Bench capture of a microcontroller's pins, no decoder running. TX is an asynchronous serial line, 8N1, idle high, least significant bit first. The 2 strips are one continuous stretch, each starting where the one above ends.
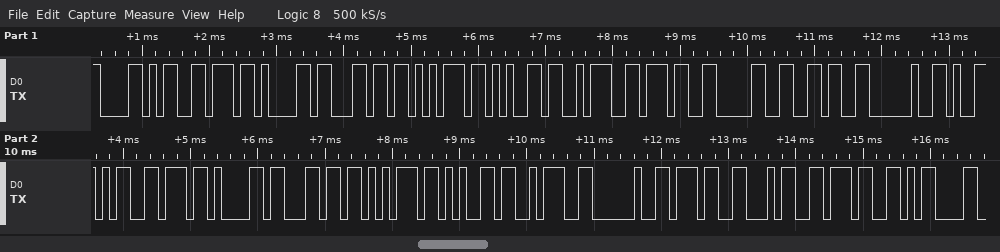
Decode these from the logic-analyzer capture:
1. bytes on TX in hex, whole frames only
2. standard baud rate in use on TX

58 76 61 6C 75 65 3A 37 30 36 20 59 76 61 6C 75 65 3A 20 37 34 37 0D
9600 baud
